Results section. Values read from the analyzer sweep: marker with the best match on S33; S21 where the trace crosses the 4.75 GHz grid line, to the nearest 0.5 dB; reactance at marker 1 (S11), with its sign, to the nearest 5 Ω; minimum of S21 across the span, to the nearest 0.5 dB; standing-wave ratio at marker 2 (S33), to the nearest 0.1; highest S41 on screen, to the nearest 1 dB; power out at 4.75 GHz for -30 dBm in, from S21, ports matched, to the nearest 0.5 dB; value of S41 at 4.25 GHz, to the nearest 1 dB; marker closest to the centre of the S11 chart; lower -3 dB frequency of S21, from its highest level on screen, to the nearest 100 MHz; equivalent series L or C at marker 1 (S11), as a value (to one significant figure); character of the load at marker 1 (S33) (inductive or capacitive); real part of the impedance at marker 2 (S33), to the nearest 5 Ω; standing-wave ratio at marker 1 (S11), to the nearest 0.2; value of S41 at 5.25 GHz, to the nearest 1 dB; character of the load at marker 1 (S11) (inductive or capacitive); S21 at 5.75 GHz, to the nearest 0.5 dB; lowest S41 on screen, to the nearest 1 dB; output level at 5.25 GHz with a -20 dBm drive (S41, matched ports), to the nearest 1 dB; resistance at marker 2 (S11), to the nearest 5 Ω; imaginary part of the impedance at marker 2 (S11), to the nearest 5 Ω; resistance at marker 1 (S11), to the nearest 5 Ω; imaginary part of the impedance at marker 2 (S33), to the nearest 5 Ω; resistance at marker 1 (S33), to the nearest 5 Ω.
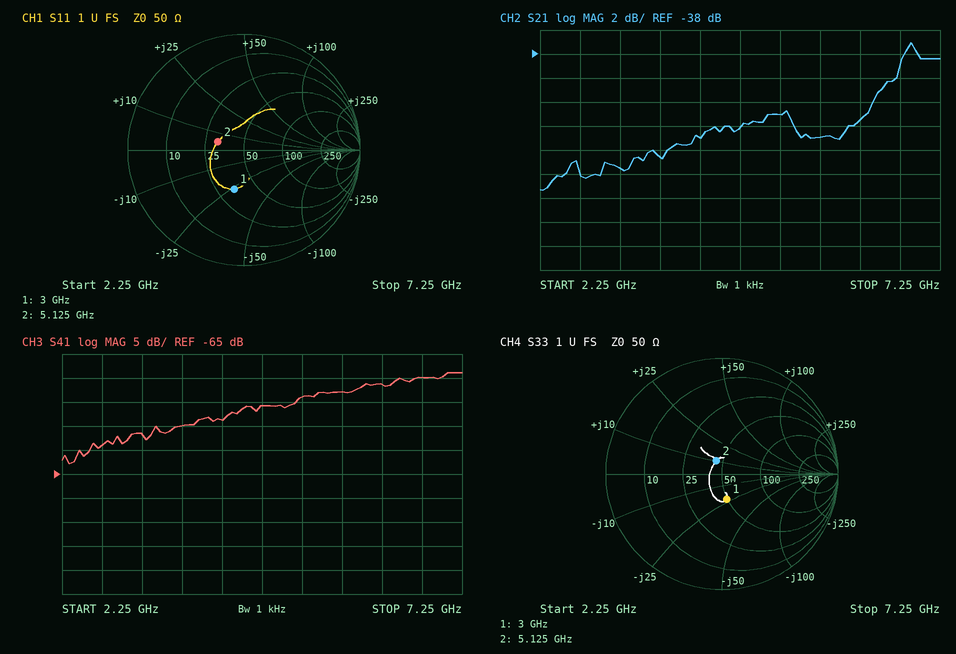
marker 2
-44.0 dB
-25 Ω
-49.5 dB
1.3
-44 dB
-74.0 dBm
-54 dB
marker 2
6.7 GHz
2 pF
capacitive
45 Ω
2.0
-49 dB
capacitive
-45.0 dB
-63 dB
-69 dBm
30 Ω
+5 Ω
35 Ω
+10 Ω
50 Ω
